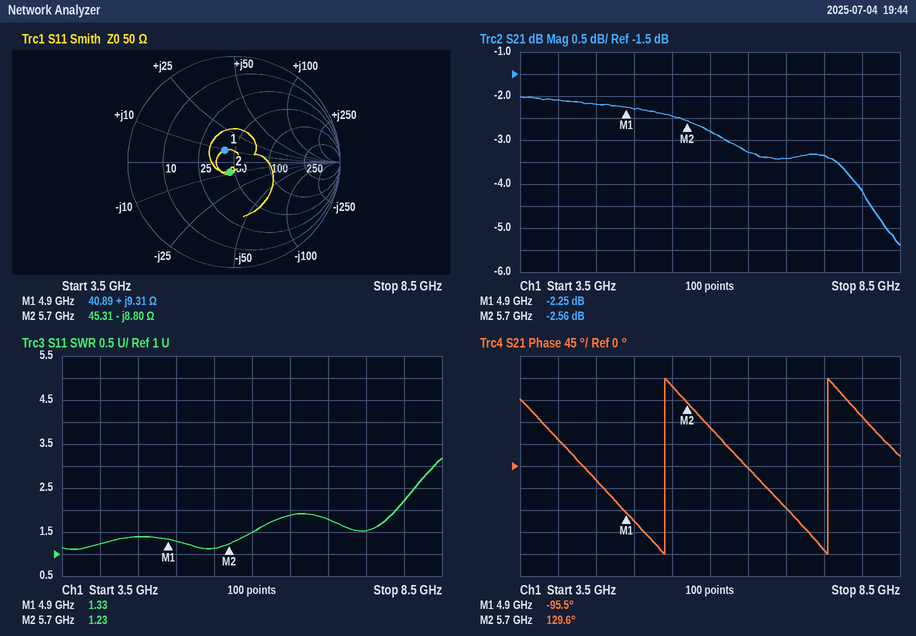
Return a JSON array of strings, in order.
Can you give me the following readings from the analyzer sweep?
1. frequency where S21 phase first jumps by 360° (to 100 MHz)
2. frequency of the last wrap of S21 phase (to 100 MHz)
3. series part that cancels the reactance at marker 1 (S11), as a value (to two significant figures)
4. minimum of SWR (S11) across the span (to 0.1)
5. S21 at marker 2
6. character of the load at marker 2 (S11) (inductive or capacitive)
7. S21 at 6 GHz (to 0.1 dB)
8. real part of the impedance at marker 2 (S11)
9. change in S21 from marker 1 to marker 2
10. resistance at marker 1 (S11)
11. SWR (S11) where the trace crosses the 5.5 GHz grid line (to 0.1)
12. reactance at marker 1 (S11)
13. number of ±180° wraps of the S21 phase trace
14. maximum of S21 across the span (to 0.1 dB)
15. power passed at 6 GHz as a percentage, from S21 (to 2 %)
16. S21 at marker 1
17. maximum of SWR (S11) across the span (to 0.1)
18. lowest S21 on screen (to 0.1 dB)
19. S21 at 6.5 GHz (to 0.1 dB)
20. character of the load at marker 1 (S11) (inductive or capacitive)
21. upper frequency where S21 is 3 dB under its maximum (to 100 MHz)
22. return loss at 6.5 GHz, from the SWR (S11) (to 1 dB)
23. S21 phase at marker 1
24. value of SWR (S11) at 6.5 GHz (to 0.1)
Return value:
["5.4 GHz", "7.5 GHz", "3.5 pF", "1.1", "-2.56 dB", "capacitive", "-2.8 dB", "45.31 Ω", "-0.31 dB", "40.89 Ω", "1.1", "+9.31 Ω", "2", "-2.0 dB", "52 %", "-2.25 dB", "3.2", "-5.4 dB", "-3.3 dB", "inductive", "8.3 GHz", "10 dB", "-95.5°", "1.9"]
